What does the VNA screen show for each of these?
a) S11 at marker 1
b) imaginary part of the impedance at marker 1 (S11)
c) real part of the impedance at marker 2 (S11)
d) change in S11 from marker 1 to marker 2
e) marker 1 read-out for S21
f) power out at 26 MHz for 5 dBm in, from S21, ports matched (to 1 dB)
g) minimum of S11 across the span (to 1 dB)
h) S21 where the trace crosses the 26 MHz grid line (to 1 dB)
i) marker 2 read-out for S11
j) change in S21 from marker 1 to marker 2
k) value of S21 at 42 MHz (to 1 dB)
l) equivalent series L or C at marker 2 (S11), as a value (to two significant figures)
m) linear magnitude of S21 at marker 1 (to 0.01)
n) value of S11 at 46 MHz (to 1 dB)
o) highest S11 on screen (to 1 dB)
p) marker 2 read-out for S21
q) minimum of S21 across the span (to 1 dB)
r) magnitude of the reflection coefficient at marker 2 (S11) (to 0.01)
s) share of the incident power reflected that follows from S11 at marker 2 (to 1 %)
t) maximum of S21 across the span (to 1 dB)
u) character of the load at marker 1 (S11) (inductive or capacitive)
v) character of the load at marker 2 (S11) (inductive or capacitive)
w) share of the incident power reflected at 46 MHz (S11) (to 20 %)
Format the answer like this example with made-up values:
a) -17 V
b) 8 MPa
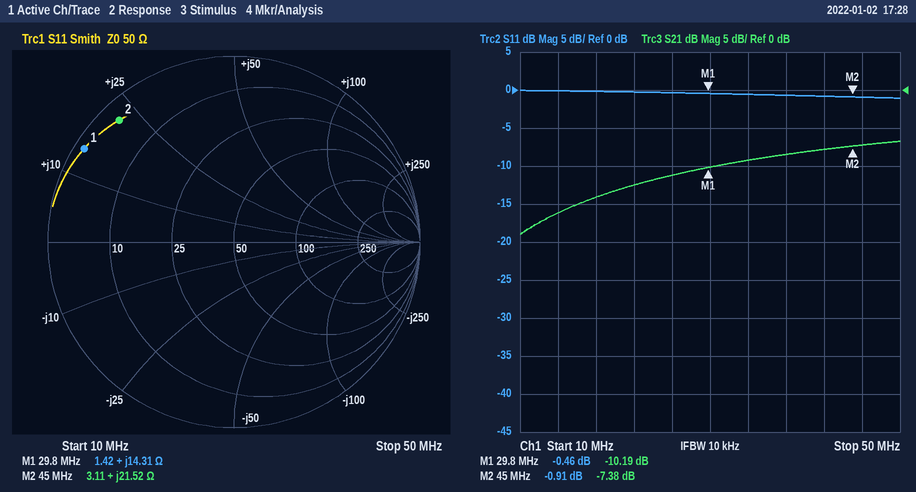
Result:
a) -0.46 dB
b) +14.31 Ω
c) 3.11 Ω
d) -0.45 dB
e) -10.19 dB
f) -6 dBm
g) -1 dB
h) -11 dB
i) -0.91 dB
j) 2.81 dB
k) -8 dB
l) 76 nH
m) 0.31
n) -1 dB
o) 0 dB
p) -7.38 dB
q) -19 dB
r) 0.90
s) 81 %
t) -7 dB
u) inductive
v) inductive
w) 80 %
